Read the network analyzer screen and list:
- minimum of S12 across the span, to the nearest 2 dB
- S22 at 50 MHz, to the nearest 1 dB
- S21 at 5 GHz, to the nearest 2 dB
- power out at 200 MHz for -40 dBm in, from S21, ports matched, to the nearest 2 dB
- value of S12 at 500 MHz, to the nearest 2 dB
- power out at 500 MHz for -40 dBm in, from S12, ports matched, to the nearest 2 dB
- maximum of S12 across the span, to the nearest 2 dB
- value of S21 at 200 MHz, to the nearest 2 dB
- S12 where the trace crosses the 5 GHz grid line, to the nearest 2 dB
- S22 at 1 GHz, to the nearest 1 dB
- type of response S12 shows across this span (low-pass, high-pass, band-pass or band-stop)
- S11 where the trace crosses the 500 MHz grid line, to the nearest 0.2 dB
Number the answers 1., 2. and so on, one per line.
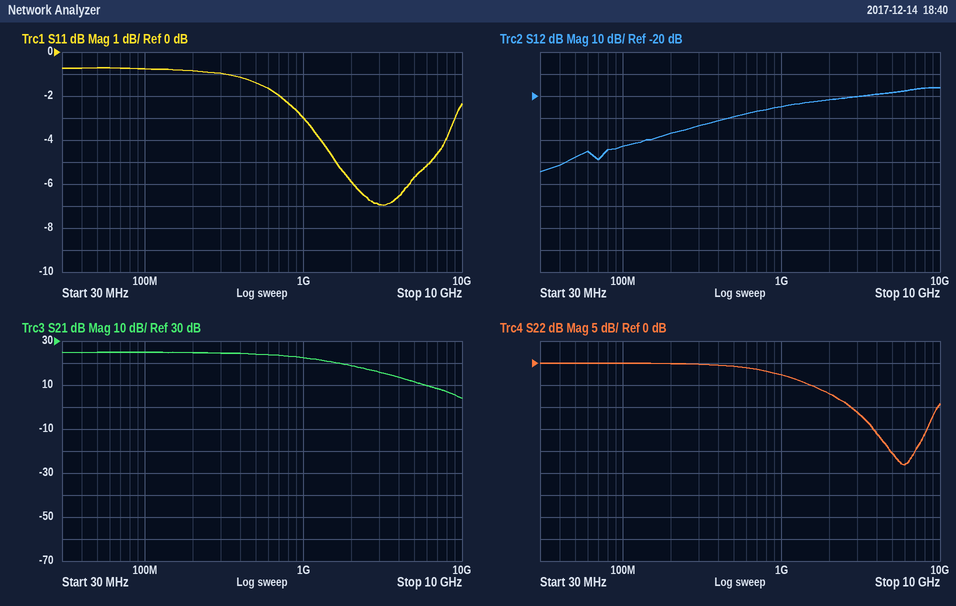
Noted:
1. -54 dB
2. 0 dB
3. 12 dB
4. -16 dBm
5. -30 dB
6. -70 dBm
7. -16 dB
8. 24 dB
9. -18 dB
10. -3 dB
11. high-pass
12. -1.4 dB
